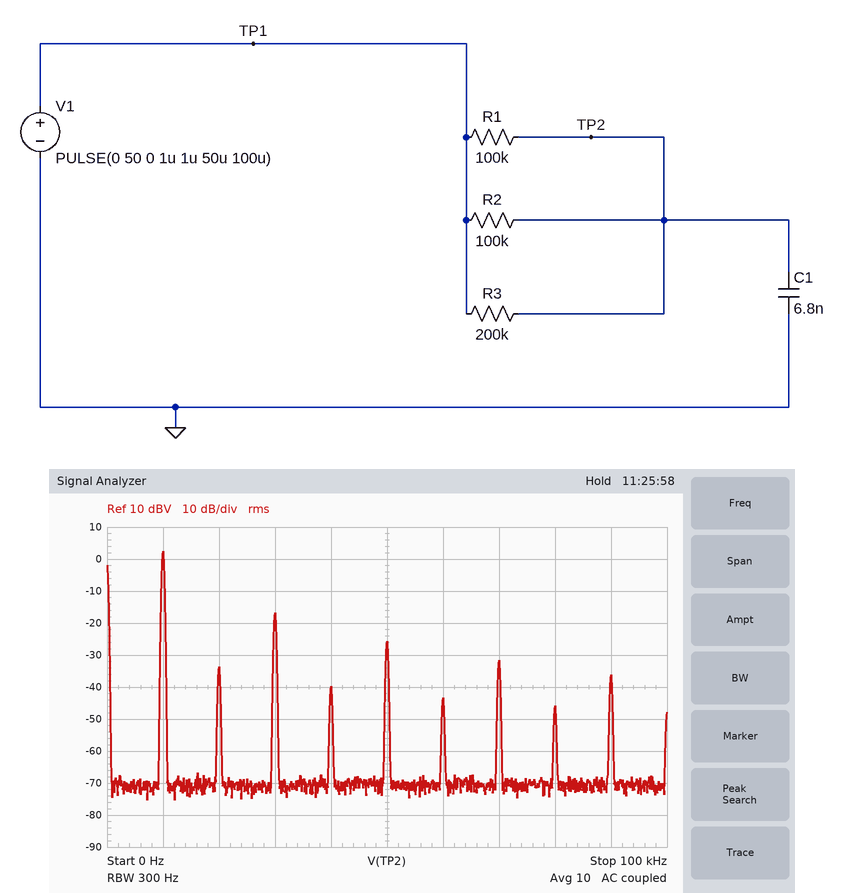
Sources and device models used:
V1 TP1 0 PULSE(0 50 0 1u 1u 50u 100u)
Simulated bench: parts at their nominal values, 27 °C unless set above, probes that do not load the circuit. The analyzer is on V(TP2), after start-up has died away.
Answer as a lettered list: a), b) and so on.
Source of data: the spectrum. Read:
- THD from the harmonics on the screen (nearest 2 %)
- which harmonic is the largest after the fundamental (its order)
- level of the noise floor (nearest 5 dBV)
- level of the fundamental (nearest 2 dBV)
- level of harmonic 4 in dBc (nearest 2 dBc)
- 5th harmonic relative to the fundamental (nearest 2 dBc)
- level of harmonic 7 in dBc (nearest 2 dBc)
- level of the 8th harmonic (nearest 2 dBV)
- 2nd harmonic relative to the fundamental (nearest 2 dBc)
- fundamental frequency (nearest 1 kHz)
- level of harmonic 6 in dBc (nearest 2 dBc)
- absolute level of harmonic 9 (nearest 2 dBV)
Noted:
a) 12 %
b) 3
c) -70 dBV
d) 2 dBV
e) -42 dBc
f) -28 dBc
g) -34 dBc
h) -46 dBV
i) -36 dBc
j) 10 kHz
k) -46 dBc
l) -36 dBV
